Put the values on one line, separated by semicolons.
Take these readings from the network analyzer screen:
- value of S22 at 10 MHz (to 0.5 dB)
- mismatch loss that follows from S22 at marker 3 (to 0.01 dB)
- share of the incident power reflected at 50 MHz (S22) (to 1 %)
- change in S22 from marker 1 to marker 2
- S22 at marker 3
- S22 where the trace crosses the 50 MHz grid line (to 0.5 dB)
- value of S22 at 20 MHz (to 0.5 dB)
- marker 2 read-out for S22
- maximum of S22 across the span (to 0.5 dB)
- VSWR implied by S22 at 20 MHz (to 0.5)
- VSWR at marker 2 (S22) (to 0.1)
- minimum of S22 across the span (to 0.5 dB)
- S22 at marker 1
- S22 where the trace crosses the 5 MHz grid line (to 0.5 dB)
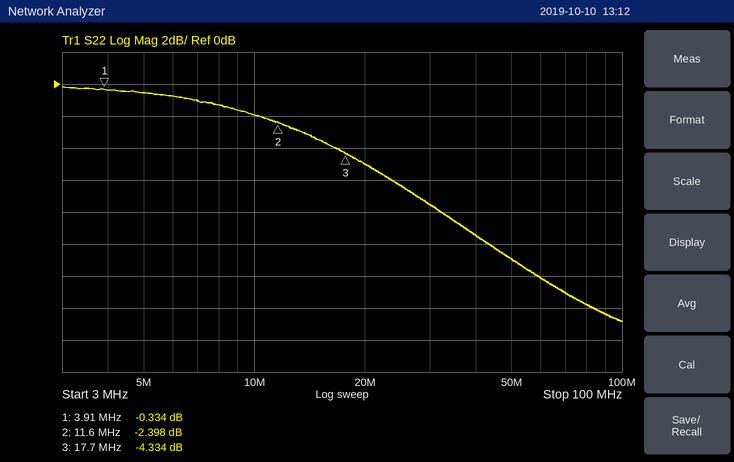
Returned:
-2.0 dB; 2.00 dB; 8 %; -2.064 dB; -4.334 dB; -11.0 dB; -5.0 dB; -2.398 dB; 0.0 dB; 3.5; 7.3; -15.0 dB; -0.334 dB; -0.5 dB
